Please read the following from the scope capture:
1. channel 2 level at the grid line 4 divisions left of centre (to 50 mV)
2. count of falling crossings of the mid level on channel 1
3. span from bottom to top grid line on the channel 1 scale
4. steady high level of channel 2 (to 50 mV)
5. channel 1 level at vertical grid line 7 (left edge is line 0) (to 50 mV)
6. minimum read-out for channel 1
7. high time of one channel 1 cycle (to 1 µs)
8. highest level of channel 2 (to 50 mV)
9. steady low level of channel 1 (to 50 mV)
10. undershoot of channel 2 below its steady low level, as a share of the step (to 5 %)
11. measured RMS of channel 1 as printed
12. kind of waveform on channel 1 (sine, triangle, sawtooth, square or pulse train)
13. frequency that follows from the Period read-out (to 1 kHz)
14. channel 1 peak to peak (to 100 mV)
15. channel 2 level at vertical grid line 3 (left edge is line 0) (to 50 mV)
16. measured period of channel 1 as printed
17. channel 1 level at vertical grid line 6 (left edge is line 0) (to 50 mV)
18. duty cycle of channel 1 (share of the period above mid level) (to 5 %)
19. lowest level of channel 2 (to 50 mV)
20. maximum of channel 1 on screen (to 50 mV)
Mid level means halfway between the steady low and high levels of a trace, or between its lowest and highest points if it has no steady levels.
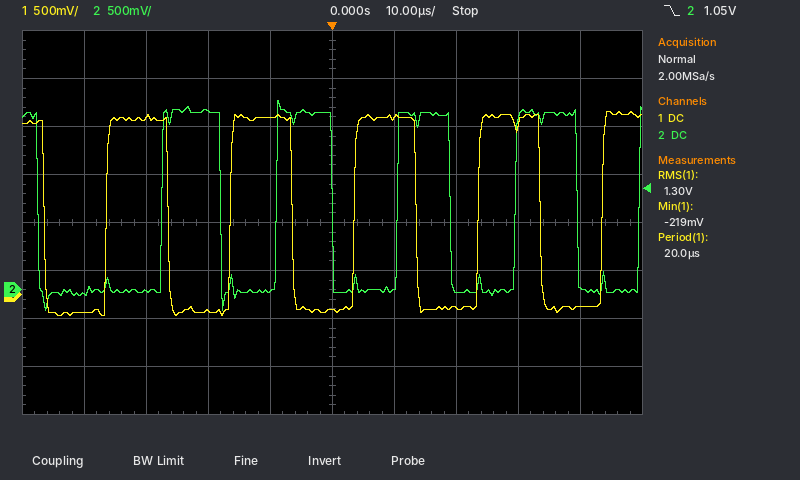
-50 mV
5
4 V
1.85 V
-150 mV
-219 mV
10 µs
1.95 V
-150 mV
10 %
1.30 V
square
50 kHz
2.10 V
1.85 V
20.0 µs
1.85 V
50 %
-200 mV
1.90 V
